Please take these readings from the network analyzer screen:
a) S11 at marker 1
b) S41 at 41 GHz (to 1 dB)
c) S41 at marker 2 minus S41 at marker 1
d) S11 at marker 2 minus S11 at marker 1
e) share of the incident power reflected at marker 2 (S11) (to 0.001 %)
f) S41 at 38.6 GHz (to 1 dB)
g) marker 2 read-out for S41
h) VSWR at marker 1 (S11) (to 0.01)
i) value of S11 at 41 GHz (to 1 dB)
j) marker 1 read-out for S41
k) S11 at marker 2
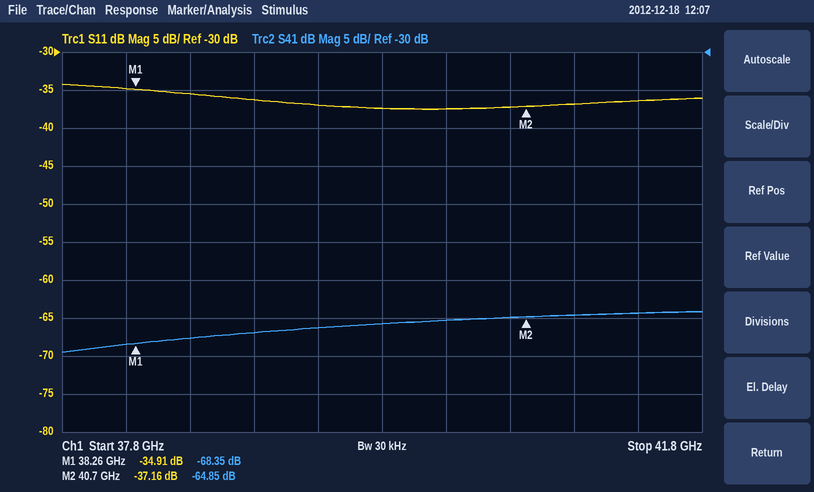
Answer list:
-34.91 dB
-65 dB
3.50 dB
-2.25 dB
0.019 %
-68 dB
-64.85 dB
1.04
-37 dB
-68.35 dB
-37.16 dB
